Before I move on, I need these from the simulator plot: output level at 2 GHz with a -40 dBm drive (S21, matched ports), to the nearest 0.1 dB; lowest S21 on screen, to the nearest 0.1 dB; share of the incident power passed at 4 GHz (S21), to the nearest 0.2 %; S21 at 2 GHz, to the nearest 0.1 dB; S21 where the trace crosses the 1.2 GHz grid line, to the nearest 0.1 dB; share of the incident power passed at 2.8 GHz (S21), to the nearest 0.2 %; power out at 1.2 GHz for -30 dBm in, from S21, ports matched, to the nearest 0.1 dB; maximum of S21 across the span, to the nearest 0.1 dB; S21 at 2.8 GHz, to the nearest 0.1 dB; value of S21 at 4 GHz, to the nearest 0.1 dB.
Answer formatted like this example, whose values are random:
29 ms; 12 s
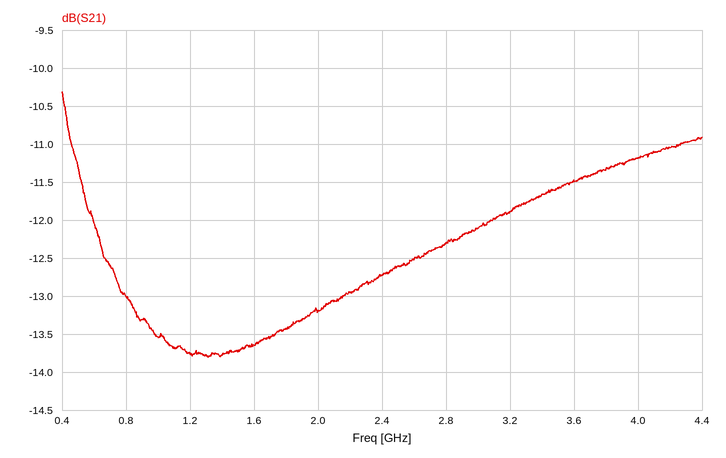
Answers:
-53.2 dBm; -13.8 dB; 7.6 %; -13.2 dB; -13.8 dB; 5.8 %; -43.8 dBm; -10.3 dB; -12.3 dB; -11.2 dB
